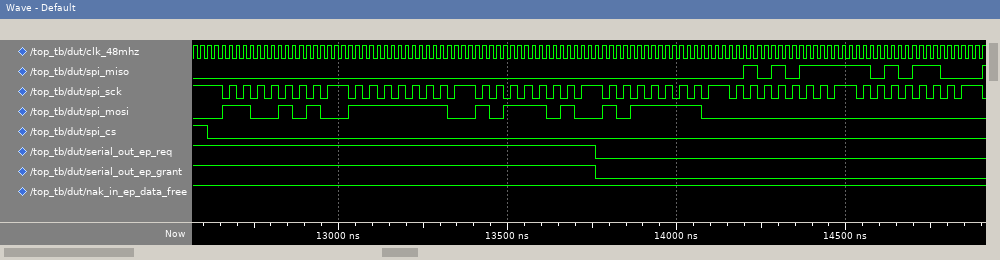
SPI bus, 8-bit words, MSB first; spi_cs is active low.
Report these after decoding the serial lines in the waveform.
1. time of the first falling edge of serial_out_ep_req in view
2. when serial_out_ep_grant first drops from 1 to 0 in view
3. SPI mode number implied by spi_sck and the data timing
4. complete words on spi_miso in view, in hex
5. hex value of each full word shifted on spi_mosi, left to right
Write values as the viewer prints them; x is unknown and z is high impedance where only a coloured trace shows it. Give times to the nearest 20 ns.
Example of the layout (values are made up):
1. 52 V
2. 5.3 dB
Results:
1. 13760 ns
2. 13760 ns
3. 3
4. 00, 00, 00, 00, 57, AC
5. CA, FE, BA, BE, 00, 00
